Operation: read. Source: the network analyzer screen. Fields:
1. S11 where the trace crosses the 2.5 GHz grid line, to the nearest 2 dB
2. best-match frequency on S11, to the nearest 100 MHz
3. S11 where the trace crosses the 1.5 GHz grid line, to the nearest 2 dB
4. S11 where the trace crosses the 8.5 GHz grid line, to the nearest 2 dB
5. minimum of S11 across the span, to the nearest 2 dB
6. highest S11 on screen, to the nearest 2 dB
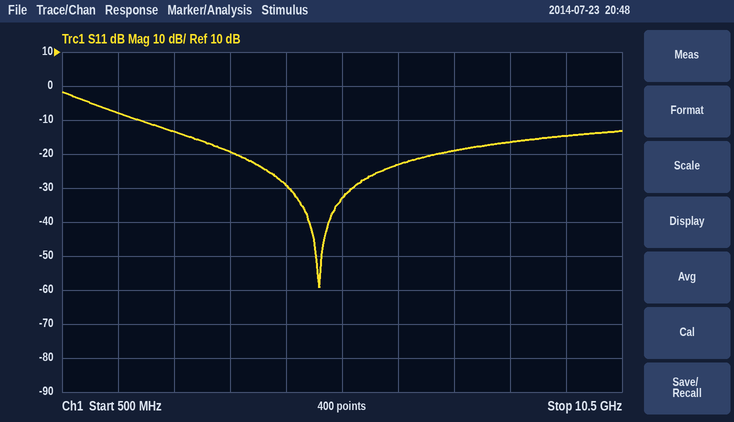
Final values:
-14 dB
5.1 GHz
-8 dB
-16 dB
-60 dB
-2 dB
